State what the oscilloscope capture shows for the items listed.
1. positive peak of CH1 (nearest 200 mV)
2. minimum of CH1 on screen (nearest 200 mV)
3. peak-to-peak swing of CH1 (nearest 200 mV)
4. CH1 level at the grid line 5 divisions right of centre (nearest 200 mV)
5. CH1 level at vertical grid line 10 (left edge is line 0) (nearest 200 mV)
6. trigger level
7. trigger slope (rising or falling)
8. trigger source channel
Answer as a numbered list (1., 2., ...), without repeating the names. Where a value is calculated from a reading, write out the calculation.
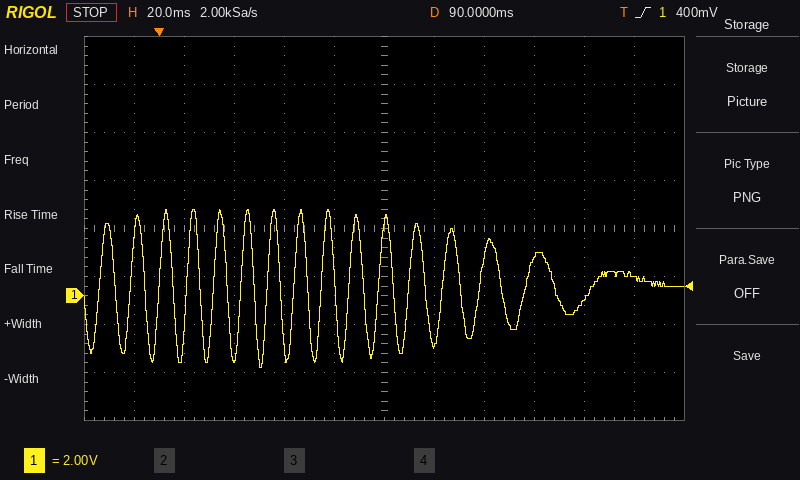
1. 3.6 V
2. -3.0 V
3. 3.6 V − (-3.0 V) = 6.6 V
4. 800 mV
5. -200 mV
6. 400 mV
7. rising
8. CH1
